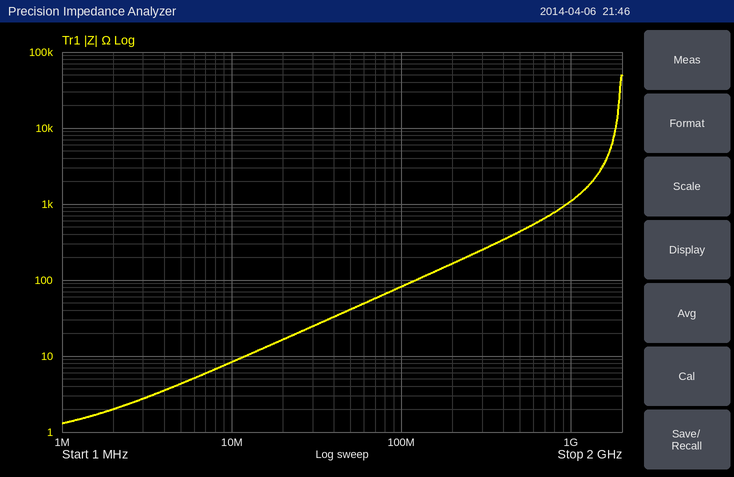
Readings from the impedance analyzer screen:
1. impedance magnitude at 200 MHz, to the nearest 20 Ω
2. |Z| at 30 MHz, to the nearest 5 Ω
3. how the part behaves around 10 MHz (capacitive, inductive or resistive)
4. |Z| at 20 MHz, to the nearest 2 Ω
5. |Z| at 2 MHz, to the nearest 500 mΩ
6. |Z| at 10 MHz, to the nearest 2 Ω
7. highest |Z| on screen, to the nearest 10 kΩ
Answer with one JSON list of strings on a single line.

["160 Ω", "25 Ω", "inductive", "16 Ω", "2.0 Ω", "8 Ω", "50 kΩ"]
